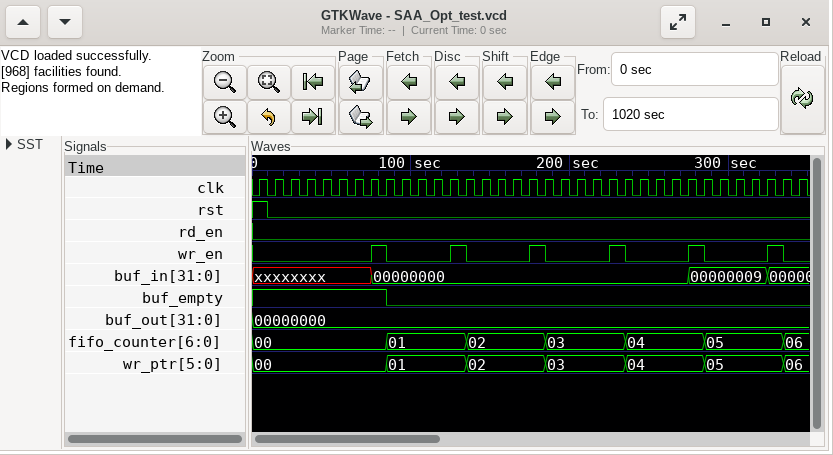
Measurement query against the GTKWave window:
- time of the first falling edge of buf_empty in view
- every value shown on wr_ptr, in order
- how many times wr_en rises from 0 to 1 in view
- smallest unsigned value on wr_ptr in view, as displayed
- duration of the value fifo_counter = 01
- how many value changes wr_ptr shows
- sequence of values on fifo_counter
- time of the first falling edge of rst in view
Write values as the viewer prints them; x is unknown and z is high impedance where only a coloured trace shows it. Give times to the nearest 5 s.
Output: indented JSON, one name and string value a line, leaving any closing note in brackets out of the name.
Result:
{
  "time of the first falling edge of buf_empty in view": "85 s",
  "every value shown on wr_ptr, in order": "00, 01, 02, 03, 04, 05, 06",
  "how many times wr_en rises from 0 to 1 in view": "6",
  "smallest unsigned value on wr_ptr in view, as displayed": "00",
  "duration of the value fifo_counter = 01": "50 s",
  "how many value changes wr_ptr shows": "6",
  "sequence of values on fifo_counter": "00, 01, 02, 03, 04, 05, 06",
  "time of the first falling edge of rst in view": "10 s"
}
